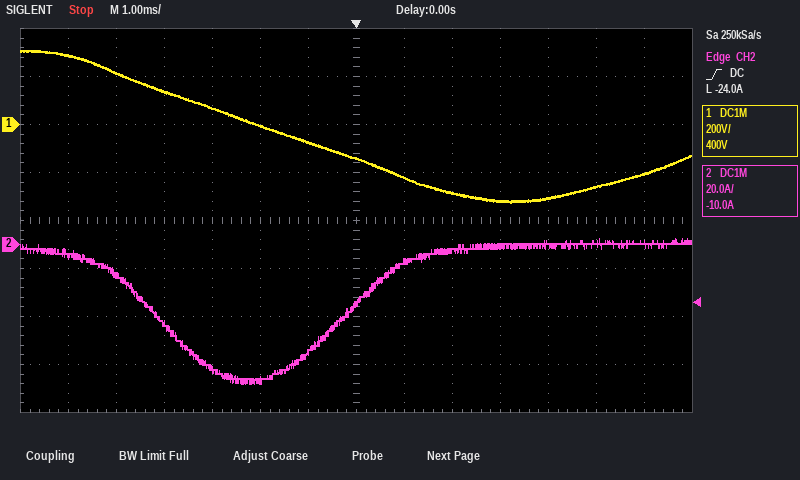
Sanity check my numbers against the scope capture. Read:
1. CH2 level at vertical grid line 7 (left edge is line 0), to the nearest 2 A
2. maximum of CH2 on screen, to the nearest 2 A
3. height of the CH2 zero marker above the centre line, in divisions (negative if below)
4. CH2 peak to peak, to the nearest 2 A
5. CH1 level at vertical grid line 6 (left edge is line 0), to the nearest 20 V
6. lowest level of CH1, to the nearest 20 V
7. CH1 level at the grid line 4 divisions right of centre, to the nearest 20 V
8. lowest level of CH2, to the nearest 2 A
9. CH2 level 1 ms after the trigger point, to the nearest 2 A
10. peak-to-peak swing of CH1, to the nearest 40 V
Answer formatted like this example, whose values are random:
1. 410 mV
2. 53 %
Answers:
1. -24 A
2. 2 A
3. -0.5 div
4. 60 A
5. -80 V
6. -320 V
7. -300 V
8. -58 A
9. -6 A
10. 640 V
